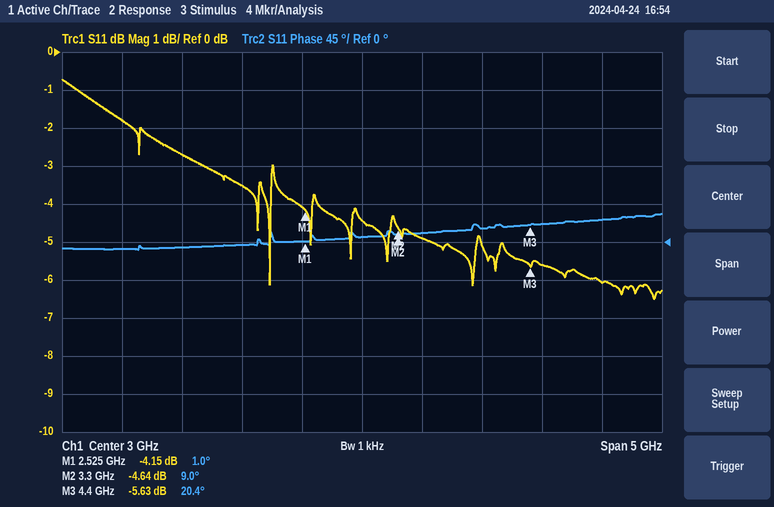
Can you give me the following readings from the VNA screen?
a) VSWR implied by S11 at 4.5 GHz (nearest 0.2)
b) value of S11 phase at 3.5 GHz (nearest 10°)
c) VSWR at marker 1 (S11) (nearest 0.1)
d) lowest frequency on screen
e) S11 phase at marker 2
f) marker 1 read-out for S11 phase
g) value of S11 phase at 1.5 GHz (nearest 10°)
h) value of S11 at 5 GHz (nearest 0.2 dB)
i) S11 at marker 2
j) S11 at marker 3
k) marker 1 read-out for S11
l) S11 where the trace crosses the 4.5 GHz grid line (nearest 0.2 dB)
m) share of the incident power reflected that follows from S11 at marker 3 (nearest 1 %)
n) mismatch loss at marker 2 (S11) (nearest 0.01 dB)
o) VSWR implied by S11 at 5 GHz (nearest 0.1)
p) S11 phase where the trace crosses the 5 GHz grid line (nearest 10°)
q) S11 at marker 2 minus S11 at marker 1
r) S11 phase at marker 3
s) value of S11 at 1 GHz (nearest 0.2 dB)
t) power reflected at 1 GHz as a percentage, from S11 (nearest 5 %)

3.2
10°
4.3
500 MHz
9.0°
1.0°
-10°
-6.0 dB
-4.64 dB
-5.63 dB
-4.15 dB
-5.6 dB
27 %
1.83 dB
3.0
30°
-0.49 dB
20.4°
-1.8 dB
65 %
